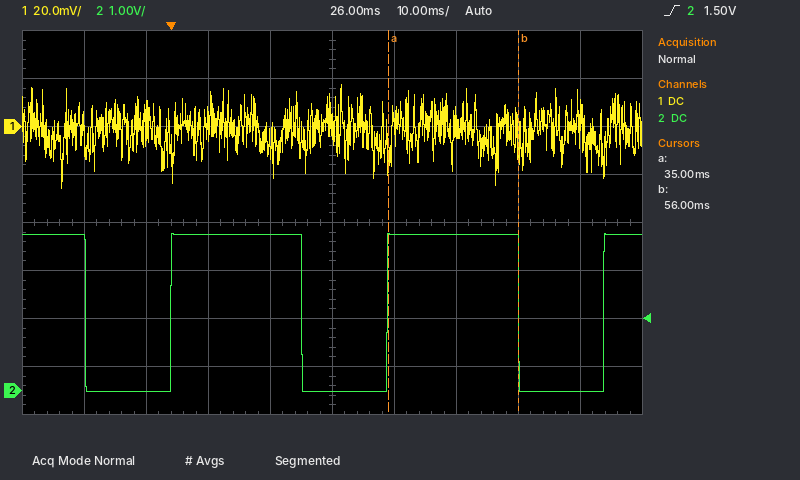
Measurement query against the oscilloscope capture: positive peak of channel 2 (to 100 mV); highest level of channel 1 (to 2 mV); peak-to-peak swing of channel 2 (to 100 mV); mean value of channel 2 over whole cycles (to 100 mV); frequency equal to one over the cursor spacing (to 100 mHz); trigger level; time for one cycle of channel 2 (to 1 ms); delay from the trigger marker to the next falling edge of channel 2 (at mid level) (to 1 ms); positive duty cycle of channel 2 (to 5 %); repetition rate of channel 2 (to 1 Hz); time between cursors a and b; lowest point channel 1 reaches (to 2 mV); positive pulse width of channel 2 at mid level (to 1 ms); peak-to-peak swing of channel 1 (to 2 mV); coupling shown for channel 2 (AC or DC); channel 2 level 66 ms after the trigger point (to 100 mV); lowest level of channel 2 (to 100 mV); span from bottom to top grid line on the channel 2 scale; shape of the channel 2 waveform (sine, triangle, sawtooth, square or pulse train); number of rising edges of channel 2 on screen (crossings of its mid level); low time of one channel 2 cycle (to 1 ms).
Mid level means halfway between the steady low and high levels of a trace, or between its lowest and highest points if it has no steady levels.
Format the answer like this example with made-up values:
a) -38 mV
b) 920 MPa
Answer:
a) 3.3 V
b) 18 mV
c) 3.3 V
d) 2.0 V
e) 47.6 Hz
f) 1.50 V
g) 35 ms
h) 21 ms
i) 60 %
j) 29 Hz
k) 21 ms
l) -26 mV
m) 21 ms
n) 44 mV
o) DC
p) 0.0 V
q) 0.0 V
r) 8 V
s) pulse train
t) 3
u) 14 ms
